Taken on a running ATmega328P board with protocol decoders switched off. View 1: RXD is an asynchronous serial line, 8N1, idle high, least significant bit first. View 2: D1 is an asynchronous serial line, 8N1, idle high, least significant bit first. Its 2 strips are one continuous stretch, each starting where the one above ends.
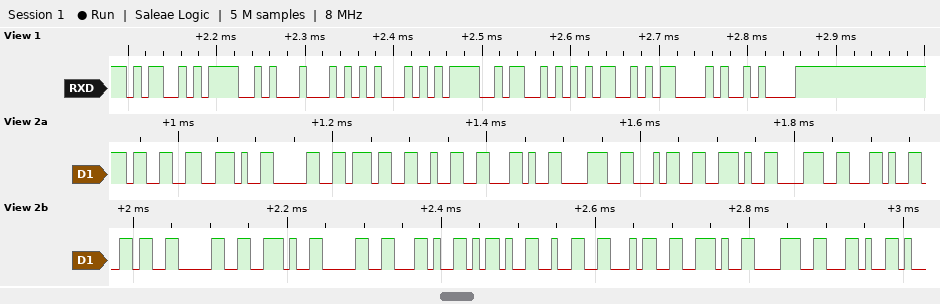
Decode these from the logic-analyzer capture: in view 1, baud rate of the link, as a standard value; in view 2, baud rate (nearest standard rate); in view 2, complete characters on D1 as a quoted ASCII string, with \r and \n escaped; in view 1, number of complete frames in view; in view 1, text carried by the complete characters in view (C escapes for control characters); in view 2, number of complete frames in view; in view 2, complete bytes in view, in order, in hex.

115200 baud
115200 baud
"3.072,84.8,60.0,-24.8,"
9
"MODE=SMC\n"
22
33 2E 30 37 32 2C 38 34 2E 38 2C 36 30 2E 30 2C 2D 32 34 2E 38 2C
